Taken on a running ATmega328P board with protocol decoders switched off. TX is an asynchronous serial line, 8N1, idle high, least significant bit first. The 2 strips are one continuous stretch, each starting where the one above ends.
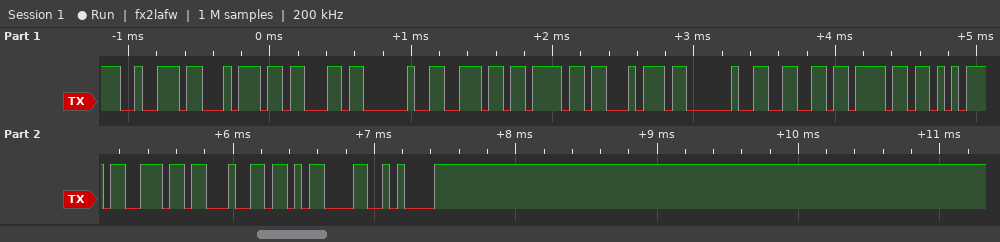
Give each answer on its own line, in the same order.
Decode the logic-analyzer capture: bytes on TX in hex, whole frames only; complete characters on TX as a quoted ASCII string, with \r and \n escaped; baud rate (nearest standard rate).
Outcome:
72 74 63 20 6E 6F 74 20 66 6F 75 6E 64 0D 0A
"rtc not found\r\n"
19200 baud
